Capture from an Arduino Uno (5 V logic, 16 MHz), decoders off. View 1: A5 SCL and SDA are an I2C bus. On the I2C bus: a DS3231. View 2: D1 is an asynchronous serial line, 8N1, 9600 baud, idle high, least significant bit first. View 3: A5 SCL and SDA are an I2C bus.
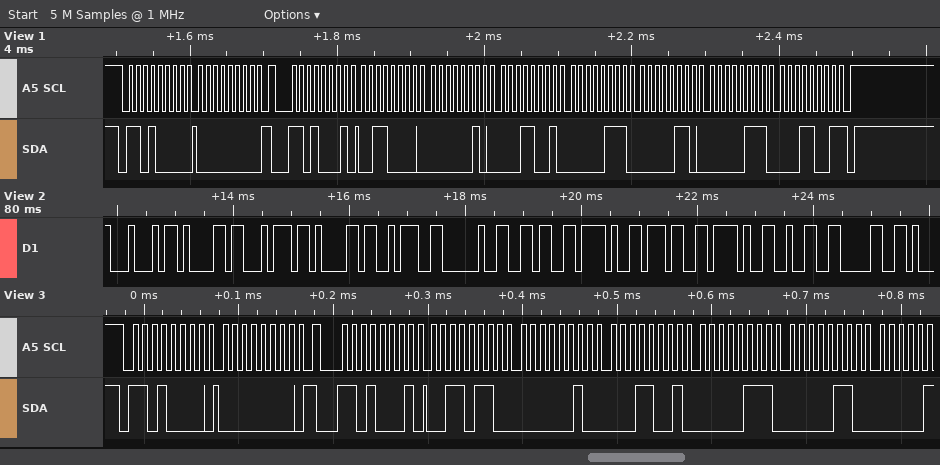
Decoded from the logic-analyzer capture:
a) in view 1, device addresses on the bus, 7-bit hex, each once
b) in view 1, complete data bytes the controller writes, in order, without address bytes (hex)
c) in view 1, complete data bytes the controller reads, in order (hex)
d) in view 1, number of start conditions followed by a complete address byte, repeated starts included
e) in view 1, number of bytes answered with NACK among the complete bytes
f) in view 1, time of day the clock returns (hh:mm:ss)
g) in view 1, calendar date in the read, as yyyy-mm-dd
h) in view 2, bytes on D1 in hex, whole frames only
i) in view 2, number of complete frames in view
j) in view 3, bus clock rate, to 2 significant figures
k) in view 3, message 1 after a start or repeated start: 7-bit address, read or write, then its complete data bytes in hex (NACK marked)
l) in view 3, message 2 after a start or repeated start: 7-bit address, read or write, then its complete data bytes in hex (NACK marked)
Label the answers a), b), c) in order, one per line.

a) 0x68
b) 00
c) 30 02 19 07 06 07 19
d) 2
e) 1
f) 19:02:30
g) 2019-07-06
h) 0x44 0x61 0x74 0x61 0x3A 0x20 0x36 0x2F 0x37 0x2F 0x32 0x30
i) 12
j) 100 kHz
k) 0x68 write: 00
l) 0x68 read: 36 02 19 07 06
